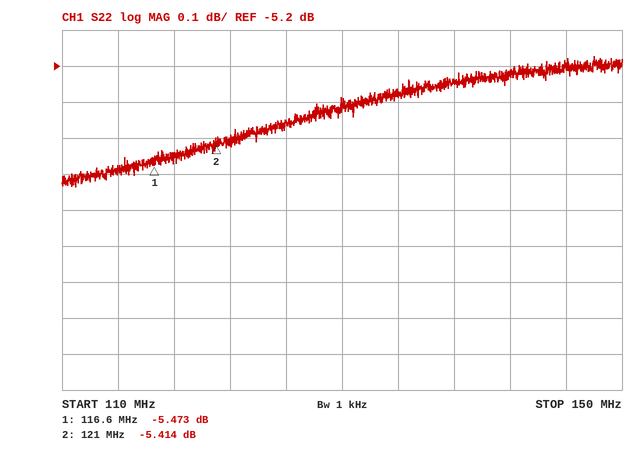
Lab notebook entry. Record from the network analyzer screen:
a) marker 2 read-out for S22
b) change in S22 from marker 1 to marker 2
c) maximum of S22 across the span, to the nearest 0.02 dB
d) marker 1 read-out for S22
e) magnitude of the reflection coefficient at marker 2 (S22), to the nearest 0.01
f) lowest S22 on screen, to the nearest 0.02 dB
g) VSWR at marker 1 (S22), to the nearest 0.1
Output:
-5.414 dB
0.059 dB
-5.18 dB
-5.473 dB
0.54
-5.54 dB
3.3
